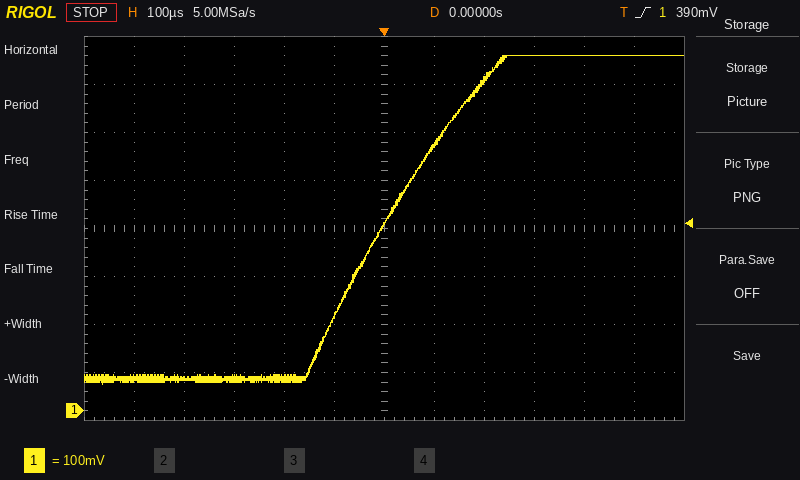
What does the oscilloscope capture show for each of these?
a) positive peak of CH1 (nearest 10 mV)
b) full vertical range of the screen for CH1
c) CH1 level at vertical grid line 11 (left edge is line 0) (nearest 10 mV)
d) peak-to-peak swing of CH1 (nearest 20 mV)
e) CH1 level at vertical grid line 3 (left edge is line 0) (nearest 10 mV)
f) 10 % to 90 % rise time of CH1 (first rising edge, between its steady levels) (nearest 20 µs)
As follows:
740 mV
800 mV
740 mV
680 mV
70 mV
320 µs
